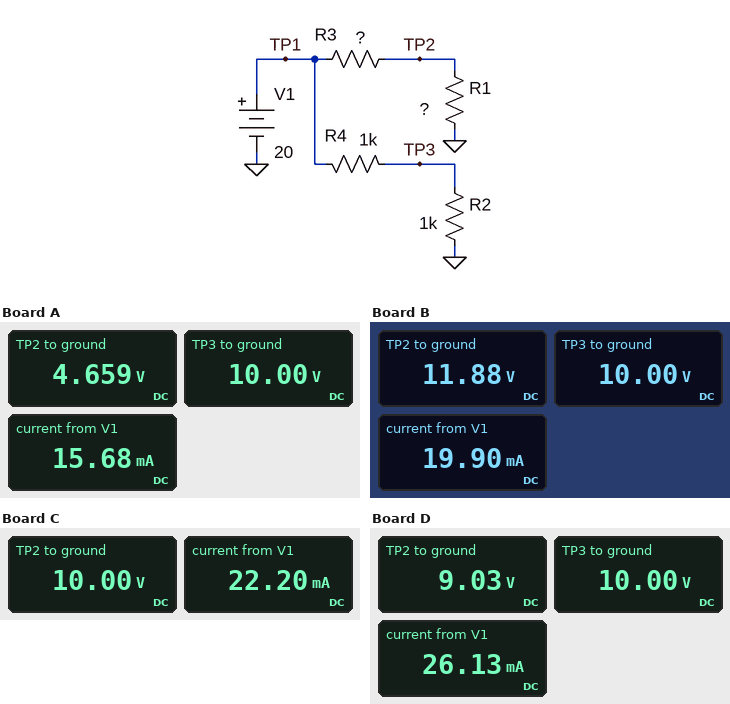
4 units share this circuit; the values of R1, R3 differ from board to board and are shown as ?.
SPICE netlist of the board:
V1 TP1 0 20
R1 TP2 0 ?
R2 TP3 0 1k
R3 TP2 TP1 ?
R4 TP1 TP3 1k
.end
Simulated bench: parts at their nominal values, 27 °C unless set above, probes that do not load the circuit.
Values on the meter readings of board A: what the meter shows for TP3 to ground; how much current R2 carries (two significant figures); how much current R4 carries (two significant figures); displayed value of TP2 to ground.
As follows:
10.00 V
10 mA
10 mA
4.659 V
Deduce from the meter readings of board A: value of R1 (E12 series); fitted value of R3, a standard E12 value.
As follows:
820 Ω
2.7 kΩ
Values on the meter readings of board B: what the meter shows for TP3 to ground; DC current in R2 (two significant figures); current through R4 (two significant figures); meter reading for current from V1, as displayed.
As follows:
10.00 V
10 mA
10 mA
19.90 mA
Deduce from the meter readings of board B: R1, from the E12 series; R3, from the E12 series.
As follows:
1.2 kΩ
820 Ω
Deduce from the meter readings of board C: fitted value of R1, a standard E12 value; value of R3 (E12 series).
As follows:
820 Ω
820 Ω
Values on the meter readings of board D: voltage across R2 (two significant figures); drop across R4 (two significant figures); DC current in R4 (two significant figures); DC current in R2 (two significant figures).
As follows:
10 V
10 V
10 mA
10 mA
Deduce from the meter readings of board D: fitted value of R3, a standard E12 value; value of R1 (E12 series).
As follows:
680 Ω
560 Ω
